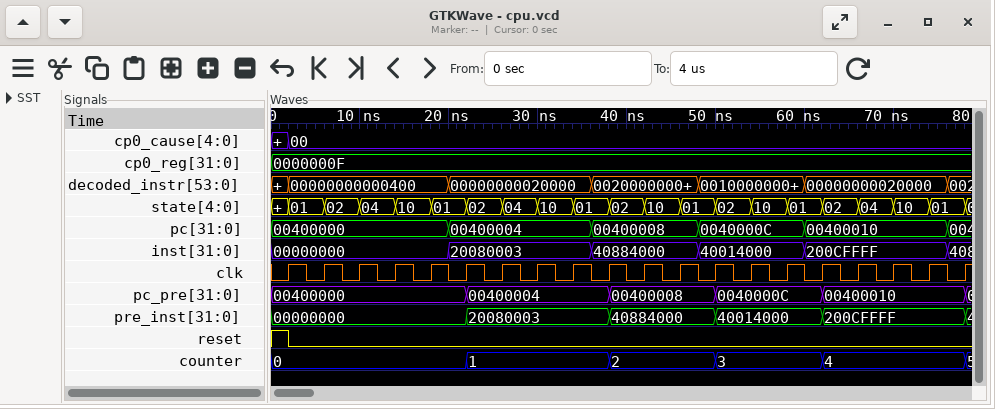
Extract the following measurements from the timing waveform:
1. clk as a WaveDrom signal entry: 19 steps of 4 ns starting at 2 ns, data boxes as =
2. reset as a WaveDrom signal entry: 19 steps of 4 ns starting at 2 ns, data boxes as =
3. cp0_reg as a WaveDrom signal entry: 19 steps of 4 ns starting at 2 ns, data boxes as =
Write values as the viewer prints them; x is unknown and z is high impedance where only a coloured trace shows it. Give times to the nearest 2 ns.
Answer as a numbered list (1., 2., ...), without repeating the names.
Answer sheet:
1. {name: 'clk', wave: 'p..................'}
2. {name: 'reset', wave: '0..................'}
3. {name: 'cp0_reg', wave: '=..................', data: '0000000F'}
